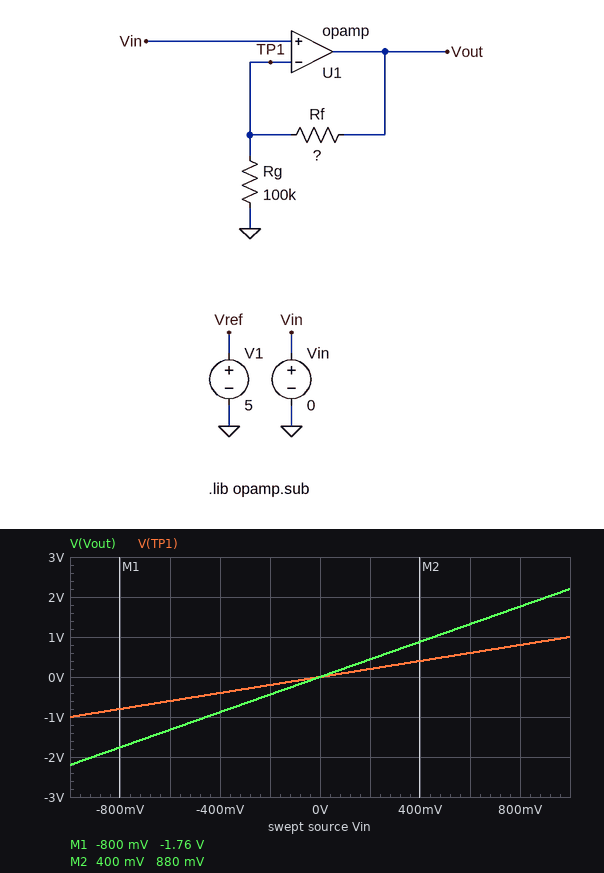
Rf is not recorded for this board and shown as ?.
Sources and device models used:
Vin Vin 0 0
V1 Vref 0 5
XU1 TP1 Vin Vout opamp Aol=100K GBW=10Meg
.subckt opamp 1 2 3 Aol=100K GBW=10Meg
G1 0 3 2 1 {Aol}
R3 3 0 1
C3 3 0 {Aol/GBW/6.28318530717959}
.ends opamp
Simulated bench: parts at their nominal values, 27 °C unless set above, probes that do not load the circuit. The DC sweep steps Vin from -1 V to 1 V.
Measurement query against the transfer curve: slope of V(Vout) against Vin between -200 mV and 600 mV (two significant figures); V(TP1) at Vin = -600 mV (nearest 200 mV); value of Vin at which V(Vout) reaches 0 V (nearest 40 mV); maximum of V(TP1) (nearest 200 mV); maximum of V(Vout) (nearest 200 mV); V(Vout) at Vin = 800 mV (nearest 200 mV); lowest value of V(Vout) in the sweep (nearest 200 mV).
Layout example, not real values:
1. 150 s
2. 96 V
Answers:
1. 2.2 V/V
2. -600 mV
3. 0 V
4. 1.0 V
5. 2.2 V
6. 1.8 V
7. -2.2 V
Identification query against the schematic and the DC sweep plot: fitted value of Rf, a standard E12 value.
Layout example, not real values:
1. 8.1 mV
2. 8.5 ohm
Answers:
1. 120 kΩ
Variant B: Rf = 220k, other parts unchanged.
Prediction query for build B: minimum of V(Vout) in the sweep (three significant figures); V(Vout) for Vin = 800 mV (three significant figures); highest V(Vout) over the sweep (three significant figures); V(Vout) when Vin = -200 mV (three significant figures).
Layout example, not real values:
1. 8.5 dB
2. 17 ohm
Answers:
1. -3.20 V
2. 2.56 V
3. 3.20 V
4. -640 mV
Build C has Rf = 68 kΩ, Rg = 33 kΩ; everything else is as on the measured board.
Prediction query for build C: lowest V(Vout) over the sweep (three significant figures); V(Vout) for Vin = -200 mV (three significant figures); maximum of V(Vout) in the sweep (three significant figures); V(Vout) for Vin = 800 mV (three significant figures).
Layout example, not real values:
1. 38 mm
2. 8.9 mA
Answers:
1. -3.06 V
2. -612 mV
3. 3.06 V
4. 2.45 V
